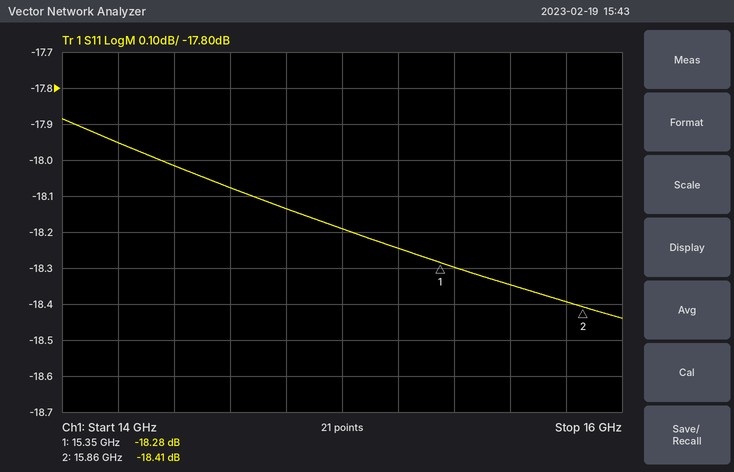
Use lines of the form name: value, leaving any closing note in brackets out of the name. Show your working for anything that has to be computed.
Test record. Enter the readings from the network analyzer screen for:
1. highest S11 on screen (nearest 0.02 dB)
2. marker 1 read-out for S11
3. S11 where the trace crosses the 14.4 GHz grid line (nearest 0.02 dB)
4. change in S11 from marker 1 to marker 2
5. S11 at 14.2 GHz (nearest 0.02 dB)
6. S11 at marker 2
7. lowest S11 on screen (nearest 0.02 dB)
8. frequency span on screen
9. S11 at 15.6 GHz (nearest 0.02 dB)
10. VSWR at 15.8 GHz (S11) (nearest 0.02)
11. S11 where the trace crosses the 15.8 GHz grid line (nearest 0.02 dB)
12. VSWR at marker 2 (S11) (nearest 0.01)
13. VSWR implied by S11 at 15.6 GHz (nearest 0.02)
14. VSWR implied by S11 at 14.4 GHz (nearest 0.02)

highest S11 on screen: -17.88 dB
marker 1 read-out for S11: -18.28 dB
S11 where the trace crosses the 14.4 GHz grid line: -18.02 dB
change in S11 from marker 1 to marker 2: -18.41 − (-18.28) = -0.13 dB
S11 at 14.2 GHz: -17.96 dB
S11 at marker 2: -18.41 dB
lowest S11 on screen: -18.44 dB
frequency span on screen: 2 GHz
S11 at 15.6 GHz: -18.34 dB
VSWR at 15.8 GHz (S11): |Γ| = 10^(-18.4/20) = 0.1202; VSWR = (1 + 0.1202)/(1 − 0.1202) ≈ 1.27, so 1.28 to the nearest 0.02
S11 where the trace crosses the 15.8 GHz grid line: -18.40 dB
VSWR at marker 2 (S11): (1 + 0.1201)/(1 − 0.1201) ≈ 1.27
VSWR implied by S11 at 15.6 GHz: |Γ| = 10^(-18.34/20) = 0.1211; VSWR = (1 + 0.1211)/(1 − 0.1211) ≈ 1.28
VSWR implied by S11 at 14.4 GHz: |Γ| = 10^(-18.02/20) = 0.1256; VSWR = (1 + 0.1256)/(1 − 0.1256) ≈ 1.29, so 1.28 to the nearest 0.02
